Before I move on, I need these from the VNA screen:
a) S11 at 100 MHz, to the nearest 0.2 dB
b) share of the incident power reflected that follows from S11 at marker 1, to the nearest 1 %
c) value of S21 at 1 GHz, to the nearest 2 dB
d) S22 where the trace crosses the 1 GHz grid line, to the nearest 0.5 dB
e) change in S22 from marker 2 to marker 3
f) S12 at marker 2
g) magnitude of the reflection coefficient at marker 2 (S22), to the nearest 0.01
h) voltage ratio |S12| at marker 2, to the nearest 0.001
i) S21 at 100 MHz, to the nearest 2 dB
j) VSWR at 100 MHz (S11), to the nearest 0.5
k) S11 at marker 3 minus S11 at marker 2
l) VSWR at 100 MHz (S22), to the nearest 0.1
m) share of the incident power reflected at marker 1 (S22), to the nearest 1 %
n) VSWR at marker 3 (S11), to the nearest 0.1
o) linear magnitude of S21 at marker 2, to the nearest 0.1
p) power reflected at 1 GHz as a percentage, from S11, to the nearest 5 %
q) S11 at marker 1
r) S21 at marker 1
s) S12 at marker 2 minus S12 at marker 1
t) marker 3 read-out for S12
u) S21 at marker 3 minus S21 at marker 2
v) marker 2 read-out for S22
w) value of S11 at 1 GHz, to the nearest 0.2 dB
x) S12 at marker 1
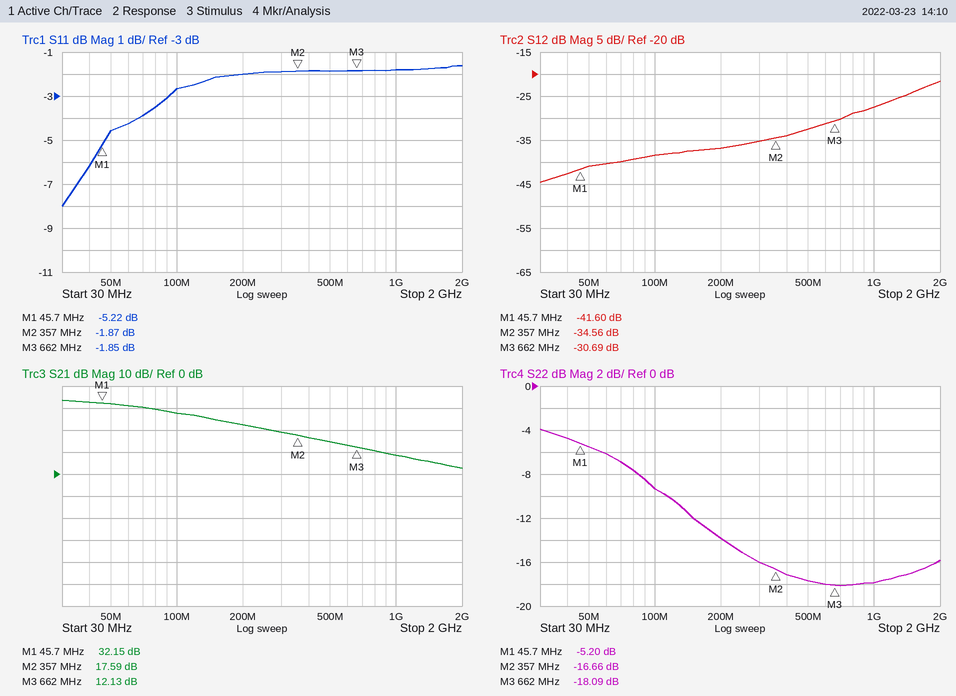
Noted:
-2.6 dB
30 %
8 dB
-18.0 dB
-1.43 dB
-34.56 dB
0.15
0.019
28 dB
6.5
0.02 dB
2.0
30 %
9.4
7.6
65 %
-5.22 dB
32.15 dB
7.04 dB
-30.69 dB
-5.46 dB
-16.66 dB
-1.8 dB
-41.60 dB
